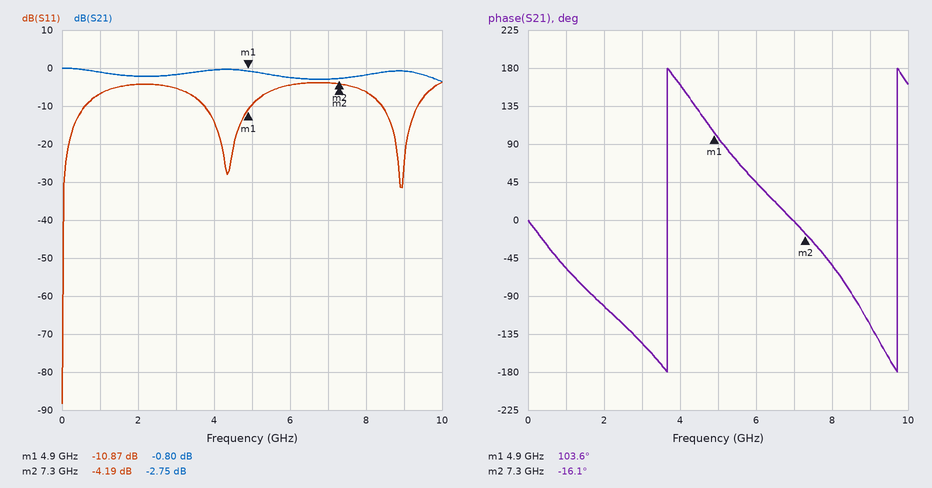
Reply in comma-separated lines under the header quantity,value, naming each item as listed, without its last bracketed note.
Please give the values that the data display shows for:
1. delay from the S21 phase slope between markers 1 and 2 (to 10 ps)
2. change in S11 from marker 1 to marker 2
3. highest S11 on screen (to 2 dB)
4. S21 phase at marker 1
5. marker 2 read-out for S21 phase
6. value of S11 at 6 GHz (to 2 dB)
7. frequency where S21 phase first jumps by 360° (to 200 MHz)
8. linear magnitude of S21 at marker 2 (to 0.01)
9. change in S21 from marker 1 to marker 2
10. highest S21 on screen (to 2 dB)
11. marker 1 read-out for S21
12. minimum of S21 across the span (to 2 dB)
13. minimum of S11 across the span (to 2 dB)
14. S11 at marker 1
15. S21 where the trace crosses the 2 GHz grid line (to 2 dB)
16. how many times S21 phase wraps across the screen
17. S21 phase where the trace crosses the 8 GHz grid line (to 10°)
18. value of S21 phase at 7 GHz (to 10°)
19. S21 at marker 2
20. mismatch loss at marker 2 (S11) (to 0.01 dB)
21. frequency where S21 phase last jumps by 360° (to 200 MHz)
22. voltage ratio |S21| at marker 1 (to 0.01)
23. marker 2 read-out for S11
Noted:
quantity,value
delay from the S21 phase slope between markers 1 and 2,140 ps
change in S11 from marker 1 to marker 2,6.68 dB
highest S11 on screen,-4 dB
S21 phase at marker 1,103.6°
marker 2 read-out for S21 phase,-16.1°
value of S11 at 6 GHz,-4 dB
frequency where S21 phase first jumps by 360°,3.6 GHz
linear magnitude of S21 at marker 2,0.73
change in S21 from marker 1 to marker 2,-1.95 dB
highest S21 on screen,0 dB
marker 1 read-out for S21,-0.80 dB
minimum of S21 across the span,-4 dB
minimum of S11 across the span,-88 dB
S11 at marker 1,-10.87 dB
S21 where the trace crosses the 2 GHz grid line,-2 dB
how many times S21 phase wraps across the screen,2
S21 phase where the trace crosses the 8 GHz grid line,-50°
value of S21 phase at 7 GHz,0°
S21 at marker 2,-2.75 dB
mismatch loss at marker 2 (S11),2.08 dB
frequency where S21 phase last jumps by 360°,9.8 GHz
voltage ratio |S21| at marker 1,0.91
marker 2 read-out for S11,-4.19 dB
